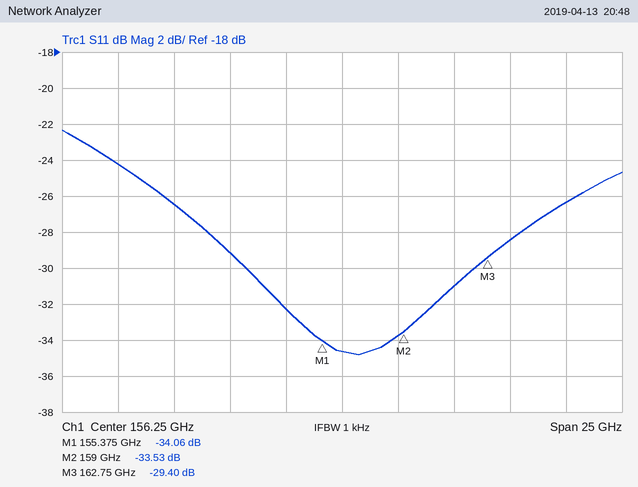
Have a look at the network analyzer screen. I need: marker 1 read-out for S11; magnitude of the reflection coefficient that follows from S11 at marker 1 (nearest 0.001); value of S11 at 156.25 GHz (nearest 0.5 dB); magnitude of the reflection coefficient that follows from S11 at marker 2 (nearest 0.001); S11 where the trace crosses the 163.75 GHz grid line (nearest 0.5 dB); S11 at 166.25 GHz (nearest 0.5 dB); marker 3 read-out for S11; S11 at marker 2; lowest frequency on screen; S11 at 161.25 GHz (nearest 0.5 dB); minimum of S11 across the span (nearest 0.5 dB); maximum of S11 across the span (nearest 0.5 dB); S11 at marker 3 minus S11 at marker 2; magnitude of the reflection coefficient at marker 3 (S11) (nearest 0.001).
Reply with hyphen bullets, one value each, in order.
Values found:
- -34.06 dB
- 0.020
- -34.5 dB
- 0.021
- -28.5 dB
- -26.5 dB
- -29.40 dB
- -33.53 dB
- 143.75 GHz
- -31.0 dB
- -35.0 dB
- -22.5 dB
- 4.13 dB
- 0.034
